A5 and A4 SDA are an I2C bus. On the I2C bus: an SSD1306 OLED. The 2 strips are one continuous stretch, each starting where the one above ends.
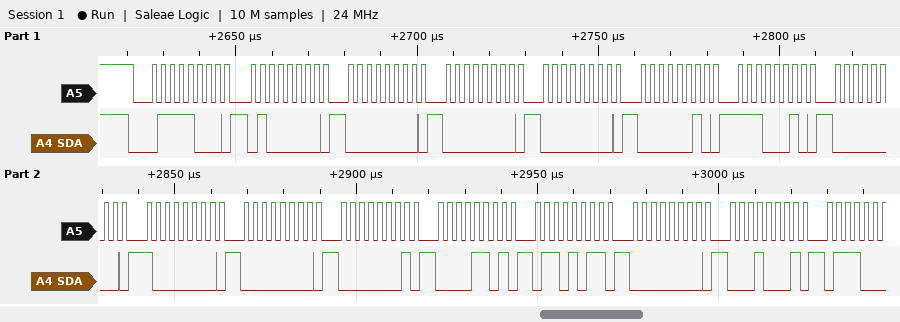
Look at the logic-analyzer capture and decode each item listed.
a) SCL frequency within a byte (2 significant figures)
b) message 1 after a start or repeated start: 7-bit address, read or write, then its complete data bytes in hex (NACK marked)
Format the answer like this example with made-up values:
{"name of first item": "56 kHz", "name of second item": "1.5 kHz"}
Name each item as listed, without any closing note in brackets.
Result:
{"SCL frequency within a byte": "400 kHz", "message 1 after a start or repeated start: 7-bit address, read or write, then its complete data bytes in hex": "0x3C write: 40 00 00 00 02 E2 00 80 00 01 0D 6B 00 11"}
